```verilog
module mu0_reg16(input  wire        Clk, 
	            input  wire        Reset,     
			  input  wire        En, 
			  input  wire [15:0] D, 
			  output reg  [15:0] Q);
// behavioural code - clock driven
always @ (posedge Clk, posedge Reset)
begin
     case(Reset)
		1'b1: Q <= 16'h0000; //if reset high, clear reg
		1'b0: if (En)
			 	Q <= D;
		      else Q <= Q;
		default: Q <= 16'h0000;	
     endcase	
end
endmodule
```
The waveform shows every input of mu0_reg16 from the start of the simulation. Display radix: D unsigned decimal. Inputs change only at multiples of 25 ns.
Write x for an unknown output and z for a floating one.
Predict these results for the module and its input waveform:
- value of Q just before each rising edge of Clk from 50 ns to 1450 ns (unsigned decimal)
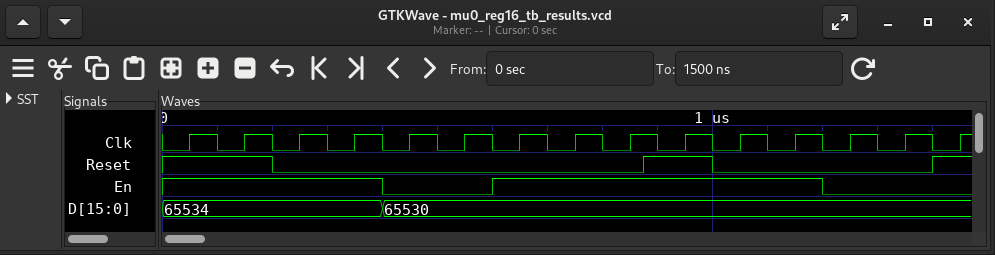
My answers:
0, 0, 0, 65534, 65534, 65534, 65534, 65530, 65530, 0, 0, 65530, 65530, 65530, 0
